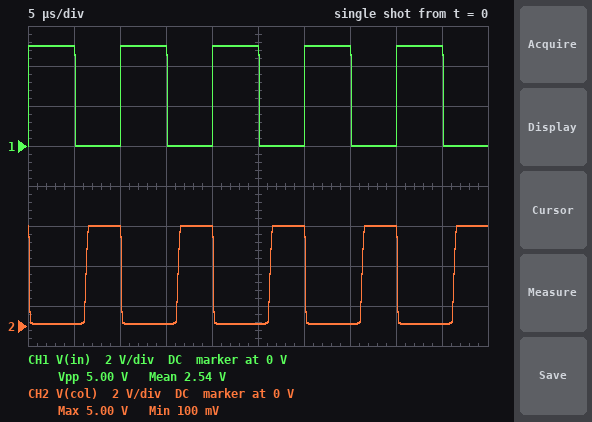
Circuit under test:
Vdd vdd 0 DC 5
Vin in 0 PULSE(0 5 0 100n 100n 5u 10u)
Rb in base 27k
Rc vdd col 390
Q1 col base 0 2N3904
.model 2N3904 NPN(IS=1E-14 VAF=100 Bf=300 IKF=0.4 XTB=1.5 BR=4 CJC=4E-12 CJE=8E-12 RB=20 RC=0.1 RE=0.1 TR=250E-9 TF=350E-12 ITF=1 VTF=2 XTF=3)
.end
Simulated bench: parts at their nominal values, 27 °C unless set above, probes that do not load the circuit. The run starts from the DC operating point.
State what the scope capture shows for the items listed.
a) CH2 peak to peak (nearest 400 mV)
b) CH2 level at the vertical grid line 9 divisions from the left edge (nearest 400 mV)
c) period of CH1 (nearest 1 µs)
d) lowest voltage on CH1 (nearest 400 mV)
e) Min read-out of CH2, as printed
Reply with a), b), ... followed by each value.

a) 4.8 V
b) 0 V
c) 10 µs
d) 0 V
e) 100 mV
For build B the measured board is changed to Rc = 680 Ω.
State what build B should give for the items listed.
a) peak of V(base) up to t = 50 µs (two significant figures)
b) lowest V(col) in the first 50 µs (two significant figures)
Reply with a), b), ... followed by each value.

a) 710 mV
b) 72 mV
